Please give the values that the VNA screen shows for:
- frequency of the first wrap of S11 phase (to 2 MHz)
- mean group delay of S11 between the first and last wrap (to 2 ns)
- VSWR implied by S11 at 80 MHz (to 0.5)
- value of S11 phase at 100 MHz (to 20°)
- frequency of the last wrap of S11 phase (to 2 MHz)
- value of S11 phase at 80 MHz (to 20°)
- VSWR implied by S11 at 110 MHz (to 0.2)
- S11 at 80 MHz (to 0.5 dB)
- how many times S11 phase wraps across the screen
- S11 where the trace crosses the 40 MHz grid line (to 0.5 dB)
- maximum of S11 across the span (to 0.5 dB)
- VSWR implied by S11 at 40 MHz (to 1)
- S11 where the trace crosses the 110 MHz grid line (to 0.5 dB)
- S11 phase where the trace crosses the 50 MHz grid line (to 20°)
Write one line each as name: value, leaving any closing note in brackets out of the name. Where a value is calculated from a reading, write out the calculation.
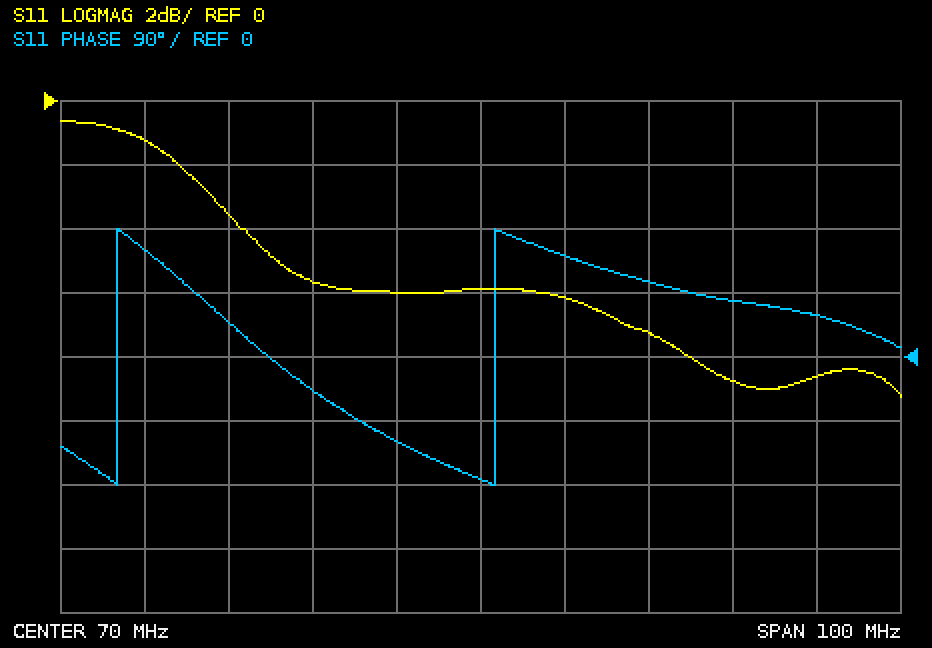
frequency of the first wrap of S11 phase: 26 MHz
mean group delay of S11 between the first and last wrap: 1 cycle / (72 MHz − 26 MHz) ≈ 22 ns
VSWR implied by S11 at 80 MHz: |Γ| = 10^(-6/20) = 0.5012; VSWR = (1 + 0.5012)/(1 − 0.5012) ≈ 3.0
value of S11 phase at 100 MHz: 80°
frequency of the last wrap of S11 phase: 72 MHz
value of S11 phase at 80 MHz: 140°
VSWR implied by S11 at 110 MHz: |Γ| = 10^(-8.5/20) = 0.3758; VSWR = (1 + 0.3758)/(1 − 0.3758) ≈ 2.2
S11 at 80 MHz: -6.0 dB
how many times S11 phase wraps across the screen: 2
S11 where the trace crosses the 40 MHz grid line: -3.5 dB
maximum of S11 across the span: -0.5 dB
VSWR implied by S11 at 40 MHz: |Γ| = 10^(-3.5/20) = 0.6683; VSWR = (1 + 0.6683)/(1 − 0.6683) ≈ 5
S11 where the trace crosses the 110 MHz grid line: -8.5 dB
S11 phase where the trace crosses the 50 MHz grid line: -40°
